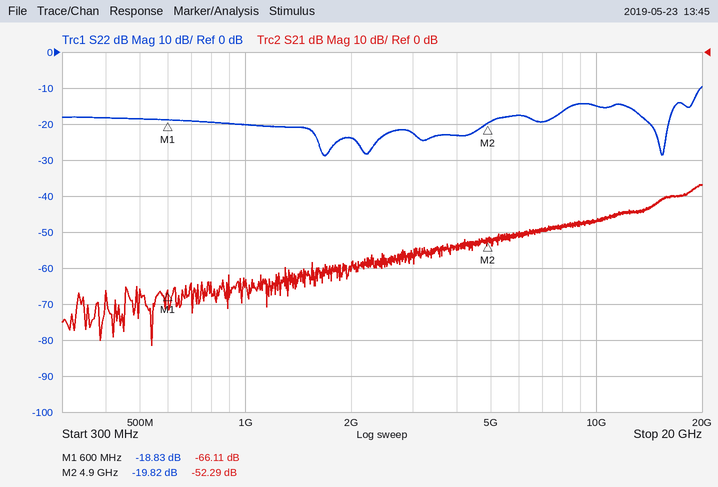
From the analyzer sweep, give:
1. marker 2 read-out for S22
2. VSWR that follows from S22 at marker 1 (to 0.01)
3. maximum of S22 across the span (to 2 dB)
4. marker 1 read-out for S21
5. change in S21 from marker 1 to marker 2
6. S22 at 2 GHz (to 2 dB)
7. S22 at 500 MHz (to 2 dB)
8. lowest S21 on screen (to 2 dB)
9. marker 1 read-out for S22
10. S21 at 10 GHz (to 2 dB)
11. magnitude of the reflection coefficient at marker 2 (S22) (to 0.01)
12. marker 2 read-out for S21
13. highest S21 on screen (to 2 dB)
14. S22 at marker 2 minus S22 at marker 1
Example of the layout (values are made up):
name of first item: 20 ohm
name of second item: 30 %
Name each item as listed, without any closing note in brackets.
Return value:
marker 2 read-out for S22: -19.82 dB
VSWR that follows from S22 at marker 1: 1.26
maximum of S22 across the span: -10 dB
marker 1 read-out for S21: -66.11 dB
change in S21 from marker 1 to marker 2: 13.82 dB
S22 at 2 GHz: -24 dB
S22 at 500 MHz: -18 dB
lowest S21 on screen: -82 dB
marker 1 read-out for S22: -18.83 dB
S21 at 10 GHz: -46 dB
magnitude of the reflection coefficient at marker 2 (S22): 0.10
marker 2 read-out for S21: -52.29 dB
highest S21 on screen: -36 dB
S22 at marker 2 minus S22 at marker 1: -0.99 dB
